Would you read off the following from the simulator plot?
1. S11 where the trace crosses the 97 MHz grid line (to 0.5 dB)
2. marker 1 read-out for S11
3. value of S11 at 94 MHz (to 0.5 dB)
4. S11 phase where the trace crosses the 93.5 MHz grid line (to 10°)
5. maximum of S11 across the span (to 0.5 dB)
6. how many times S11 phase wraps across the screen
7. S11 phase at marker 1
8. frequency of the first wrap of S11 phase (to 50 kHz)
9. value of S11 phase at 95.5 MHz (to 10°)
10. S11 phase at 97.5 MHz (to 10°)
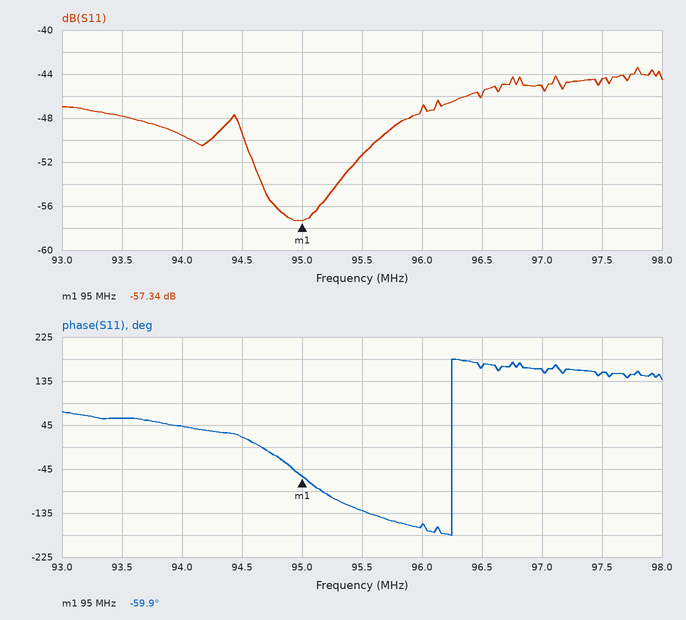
-45.0 dB
-57.34 dB
-49.5 dB
60°
-43.5 dB
1
-59.9°
96.25 MHz
-130°
150°
